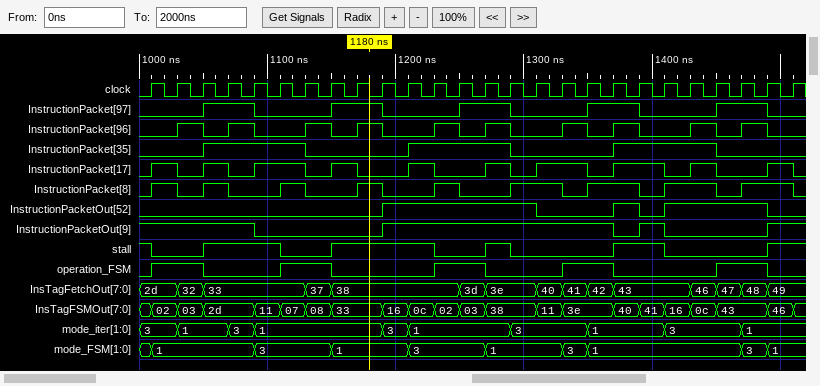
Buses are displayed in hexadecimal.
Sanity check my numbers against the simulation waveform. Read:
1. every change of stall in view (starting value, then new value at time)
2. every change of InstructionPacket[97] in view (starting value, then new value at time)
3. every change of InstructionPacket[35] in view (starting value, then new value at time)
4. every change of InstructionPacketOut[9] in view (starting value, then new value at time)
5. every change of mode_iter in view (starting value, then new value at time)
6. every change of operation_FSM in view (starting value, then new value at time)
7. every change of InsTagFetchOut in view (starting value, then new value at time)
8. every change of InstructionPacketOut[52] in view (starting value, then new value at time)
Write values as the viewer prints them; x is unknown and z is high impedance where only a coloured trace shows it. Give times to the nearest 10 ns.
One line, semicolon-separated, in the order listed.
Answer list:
1, 0 at 1010 ns, 1 at 1050 ns, 0 at 1110 ns, 1 at 1150 ns, 0 at 1230 ns, 1 at 1270 ns, 0 at 1290 ns, 1 at 1370 ns, 0 at 1410 ns, 1 at 1490 ns; 0, 1 at 1050 ns, 0 at 1090 ns, 1 at 1150 ns, 0 at 1190 ns, 1 at 1250 ns, 0 at 1290 ns, 1 at 1350 ns, 0 at 1390 ns, 1 at 1450 ns, 0 at 1490 ns; 0, 1 at 1050 ns, 0 at 1130 ns, 1 at 1210 ns, 0 at 1290 ns, 1 at 1370 ns, 0 at 1450 ns; 1, 0 at 1090 ns, 1 at 1190 ns, 0 at 1370 ns, 1 at 1390 ns, 0 at 1410 ns, 1 at 1490 ns; 3, 1 at 1030 ns, 3 at 1070 ns, 1 at 1090 ns, 3 at 1190 ns, 1 at 1210 ns, 3 at 1290 ns, 1 at 1350 ns, 3 at 1410 ns, 1 at 1470 ns; 0, 1 at 1010 ns, 0 at 1050 ns, 1 at 1110 ns, 0 at 1150 ns, 1 at 1230 ns, 0 at 1270 ns, 1 at 1330 ns, 0 at 1370 ns, 1 at 1450 ns, 0 at 1490 ns; 2d, 32 at 1030 ns, 33 at 1050 ns, 37 at 1130 ns, 38 at 1150 ns, 3d at 1250 ns, 3e at 1270 ns, 40 at 1310 ns, 41 at 1330 ns, 42 at 1350 ns, 43 at 1370 ns, 46 at 1430 ns, 47 at 1450 ns, 48 at 1470 ns, 49 at 1490 ns; 0, 1 at 1190 ns, 0 at 1310 ns, 1 at 1370 ns, 0 at 1390 ns, 1 at 1410 ns, 0 at 1490 ns
